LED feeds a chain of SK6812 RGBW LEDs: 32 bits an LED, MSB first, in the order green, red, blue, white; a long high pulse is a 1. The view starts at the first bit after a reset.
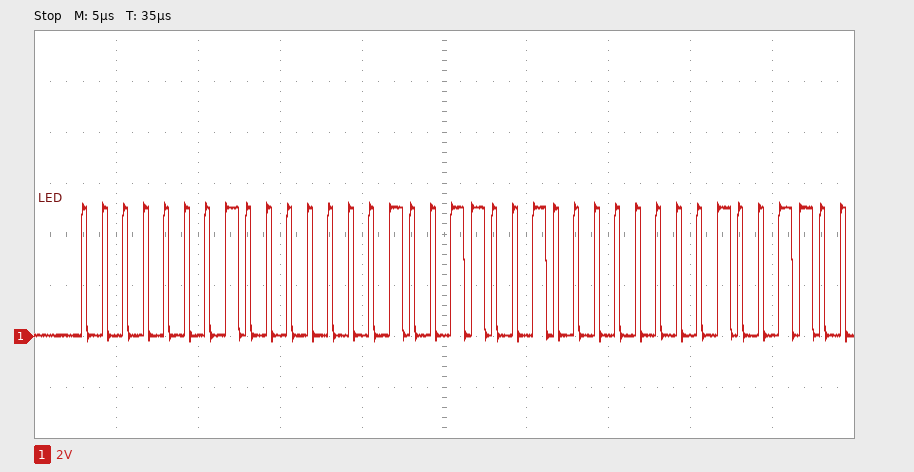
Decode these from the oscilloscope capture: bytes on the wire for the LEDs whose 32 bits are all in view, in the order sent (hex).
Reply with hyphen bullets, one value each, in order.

- 01 01 32 01
